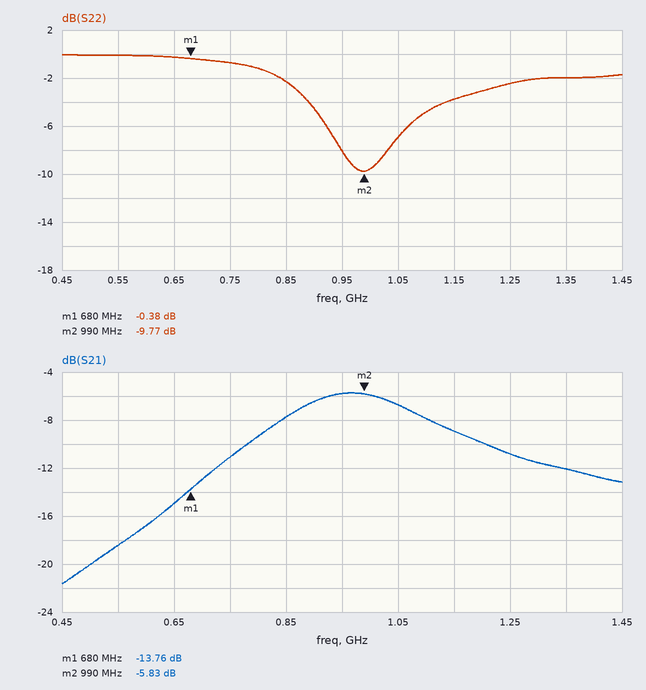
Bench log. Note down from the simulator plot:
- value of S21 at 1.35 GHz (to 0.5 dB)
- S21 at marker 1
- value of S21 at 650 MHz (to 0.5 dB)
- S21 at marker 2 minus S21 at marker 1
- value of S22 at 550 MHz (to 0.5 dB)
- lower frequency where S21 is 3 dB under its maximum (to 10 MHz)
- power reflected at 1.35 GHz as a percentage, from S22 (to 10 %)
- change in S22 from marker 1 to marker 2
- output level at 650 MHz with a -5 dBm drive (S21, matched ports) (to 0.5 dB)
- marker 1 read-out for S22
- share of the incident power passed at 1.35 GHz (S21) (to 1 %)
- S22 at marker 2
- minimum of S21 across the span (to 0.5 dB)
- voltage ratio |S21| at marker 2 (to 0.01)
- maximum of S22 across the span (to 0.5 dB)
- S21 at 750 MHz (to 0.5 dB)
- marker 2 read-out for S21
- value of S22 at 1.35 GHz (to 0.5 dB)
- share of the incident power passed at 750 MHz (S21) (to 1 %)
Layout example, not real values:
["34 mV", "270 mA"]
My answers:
["-12.0 dB", "-13.76 dB", "-15.0 dB", "7.93 dB", "0.0 dB", "820 MHz", "60 %", "-9.39 dB", "-20.0 dBm", "-0.38 dB", "6 %", "-9.77 dB", "-21.5 dB", "0.51", "0.0 dB", "-11.0 dB", "-5.83 dB", "-2.0 dB", "8 %"]
